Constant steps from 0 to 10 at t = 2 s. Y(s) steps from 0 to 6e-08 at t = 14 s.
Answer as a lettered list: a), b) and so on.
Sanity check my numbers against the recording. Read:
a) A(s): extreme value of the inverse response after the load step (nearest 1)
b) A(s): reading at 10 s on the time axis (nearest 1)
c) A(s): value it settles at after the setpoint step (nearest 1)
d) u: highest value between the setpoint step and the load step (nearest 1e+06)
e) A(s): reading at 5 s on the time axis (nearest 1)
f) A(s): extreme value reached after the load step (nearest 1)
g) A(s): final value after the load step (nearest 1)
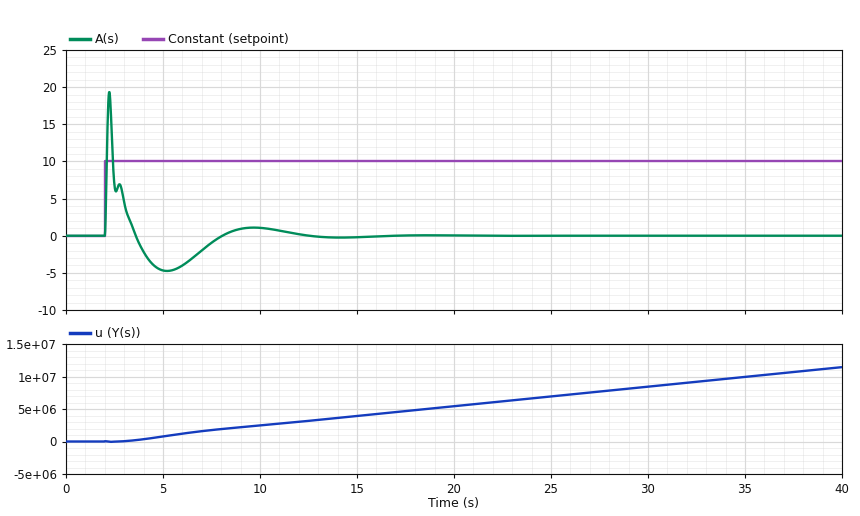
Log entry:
a) 0
b) 1
c) 0
d) 4000000
e) -5
f) 0
g) 0
